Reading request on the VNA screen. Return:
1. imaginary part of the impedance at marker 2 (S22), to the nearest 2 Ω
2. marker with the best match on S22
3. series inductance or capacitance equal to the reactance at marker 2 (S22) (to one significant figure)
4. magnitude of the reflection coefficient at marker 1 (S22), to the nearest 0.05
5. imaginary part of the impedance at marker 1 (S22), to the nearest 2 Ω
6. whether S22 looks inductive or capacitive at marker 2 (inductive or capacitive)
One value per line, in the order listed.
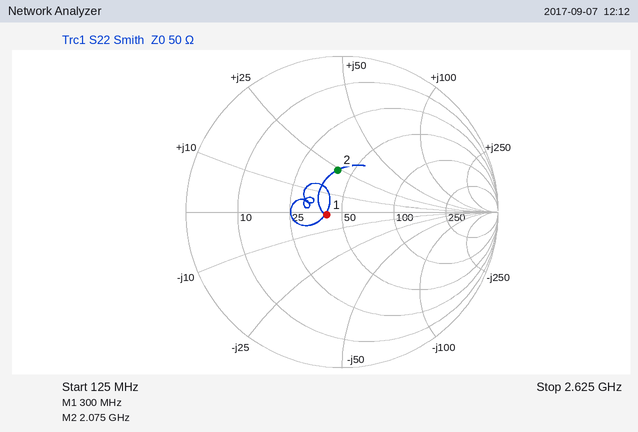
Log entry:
+24 Ω
marker 1
2 nH
0.10
-2 Ω
inductive
